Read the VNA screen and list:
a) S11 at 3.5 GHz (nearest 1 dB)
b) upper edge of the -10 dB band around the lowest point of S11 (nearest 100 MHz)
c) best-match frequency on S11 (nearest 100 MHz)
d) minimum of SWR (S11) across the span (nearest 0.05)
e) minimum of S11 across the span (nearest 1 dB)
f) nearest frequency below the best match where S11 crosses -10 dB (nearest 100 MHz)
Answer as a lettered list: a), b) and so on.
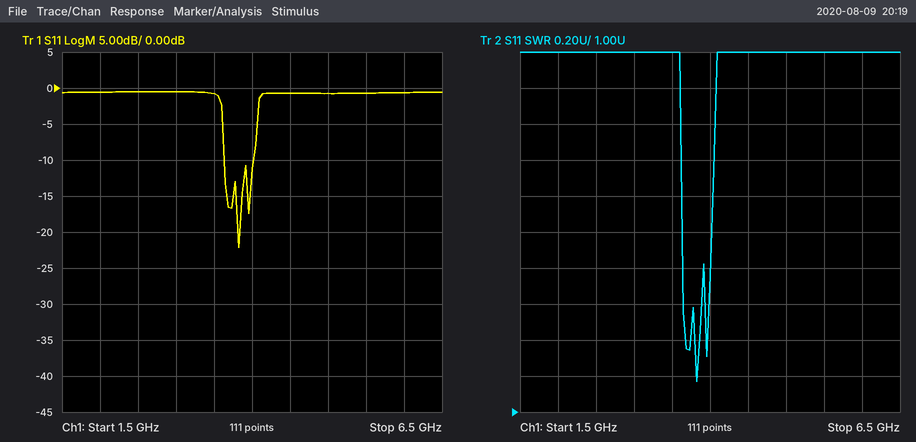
a) -1 dB
b) 4.0 GHz
c) 3.8 GHz
d) 1.15
e) -22 dB
f) 3.6 GHz
